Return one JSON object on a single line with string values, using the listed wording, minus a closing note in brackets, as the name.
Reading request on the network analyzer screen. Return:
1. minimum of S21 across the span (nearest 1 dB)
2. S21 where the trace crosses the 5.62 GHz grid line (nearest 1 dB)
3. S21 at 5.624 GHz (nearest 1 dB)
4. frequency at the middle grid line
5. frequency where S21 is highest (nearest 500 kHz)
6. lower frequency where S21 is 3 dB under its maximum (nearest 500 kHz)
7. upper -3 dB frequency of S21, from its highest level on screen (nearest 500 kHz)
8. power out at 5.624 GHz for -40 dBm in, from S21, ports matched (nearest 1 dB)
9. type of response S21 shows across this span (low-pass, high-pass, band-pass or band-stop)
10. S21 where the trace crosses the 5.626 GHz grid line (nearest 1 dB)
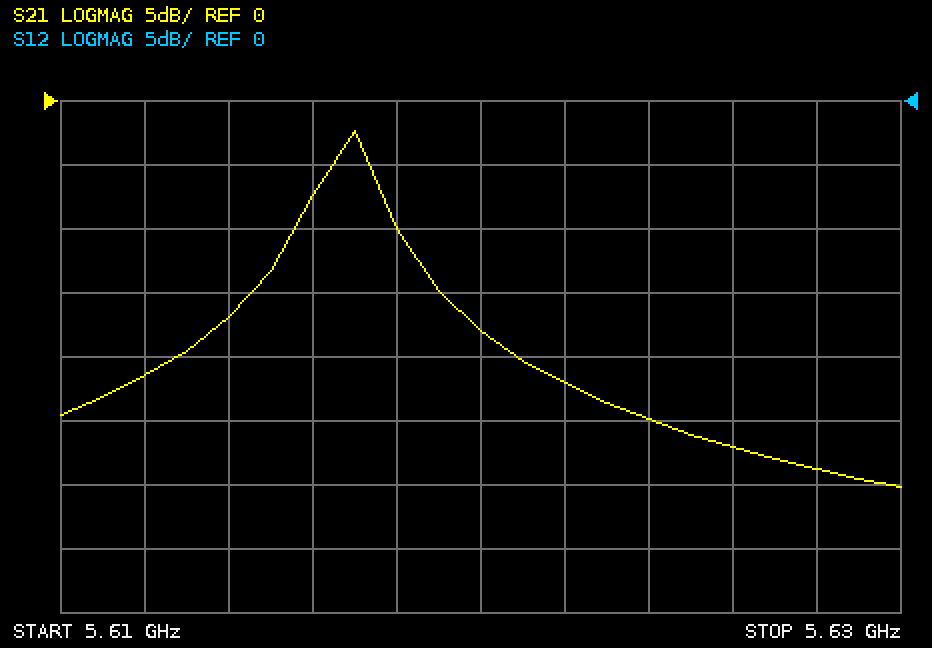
{"minimum of S21 across the span": "-30 dB", "S21 where the trace crosses the 5.62 GHz grid line": "-18 dB", "S21 at 5.624 GHz": "-25 dB", "frequency at the middle grid line": "5.62 GHz", "frequency where S21 is highest": "5.6170 GHz", "lower frequency where S21 is 3 dB under its maximum": "5.6165 GHz", "upper -3 dB frequency of S21, from its highest level on screen": "5.6175 GHz", "power out at 5.624 GHz for -40 dBm in, from S21, ports matched": "-65 dBm", "type of response S21 shows across this span": "band-pass", "S21 where the trace crosses the 5.626 GHz grid line": "-27 dB"}
